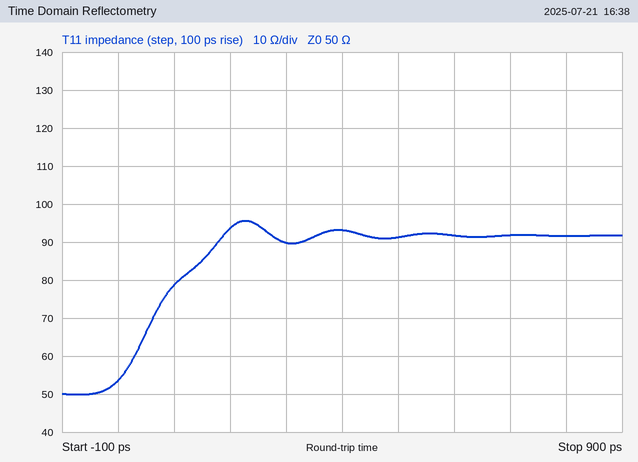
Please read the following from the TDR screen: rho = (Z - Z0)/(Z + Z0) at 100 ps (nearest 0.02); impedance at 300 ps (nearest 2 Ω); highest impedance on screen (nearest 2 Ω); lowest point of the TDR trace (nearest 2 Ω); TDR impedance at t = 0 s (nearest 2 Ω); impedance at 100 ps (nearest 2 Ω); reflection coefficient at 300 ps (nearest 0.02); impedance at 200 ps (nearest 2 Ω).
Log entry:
+0.22
90 Ω
96 Ω
50 Ω
54 Ω
78 Ω
+0.28
94 Ω
